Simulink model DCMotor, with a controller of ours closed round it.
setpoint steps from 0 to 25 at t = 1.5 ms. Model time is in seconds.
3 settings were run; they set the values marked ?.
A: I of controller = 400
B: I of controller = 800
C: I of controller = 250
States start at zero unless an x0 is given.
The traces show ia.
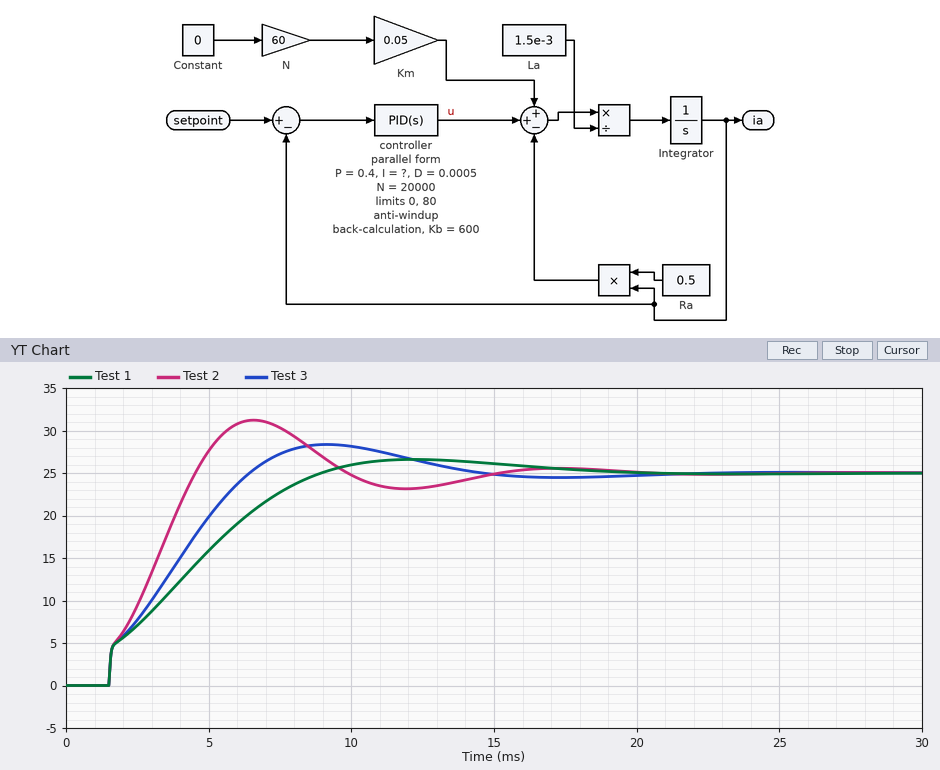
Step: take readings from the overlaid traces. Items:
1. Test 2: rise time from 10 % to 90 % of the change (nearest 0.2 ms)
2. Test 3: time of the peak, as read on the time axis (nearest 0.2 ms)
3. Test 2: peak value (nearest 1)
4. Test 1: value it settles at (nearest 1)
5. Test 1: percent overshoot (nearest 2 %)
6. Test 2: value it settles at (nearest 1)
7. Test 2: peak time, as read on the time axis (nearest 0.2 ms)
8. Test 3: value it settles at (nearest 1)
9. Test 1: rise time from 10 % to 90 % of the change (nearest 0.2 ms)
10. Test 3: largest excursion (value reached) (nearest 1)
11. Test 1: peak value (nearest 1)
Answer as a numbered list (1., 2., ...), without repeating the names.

1. 2.6 ms
2. 9.2 ms
3. 31
4. 25
5. 6 %
6. 25
7. 6.6 ms
8. 25
9. 5.8 ms
10. 28
11. 27
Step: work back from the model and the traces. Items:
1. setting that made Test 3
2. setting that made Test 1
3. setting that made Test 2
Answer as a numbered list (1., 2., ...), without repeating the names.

1. A
2. C
3. B
